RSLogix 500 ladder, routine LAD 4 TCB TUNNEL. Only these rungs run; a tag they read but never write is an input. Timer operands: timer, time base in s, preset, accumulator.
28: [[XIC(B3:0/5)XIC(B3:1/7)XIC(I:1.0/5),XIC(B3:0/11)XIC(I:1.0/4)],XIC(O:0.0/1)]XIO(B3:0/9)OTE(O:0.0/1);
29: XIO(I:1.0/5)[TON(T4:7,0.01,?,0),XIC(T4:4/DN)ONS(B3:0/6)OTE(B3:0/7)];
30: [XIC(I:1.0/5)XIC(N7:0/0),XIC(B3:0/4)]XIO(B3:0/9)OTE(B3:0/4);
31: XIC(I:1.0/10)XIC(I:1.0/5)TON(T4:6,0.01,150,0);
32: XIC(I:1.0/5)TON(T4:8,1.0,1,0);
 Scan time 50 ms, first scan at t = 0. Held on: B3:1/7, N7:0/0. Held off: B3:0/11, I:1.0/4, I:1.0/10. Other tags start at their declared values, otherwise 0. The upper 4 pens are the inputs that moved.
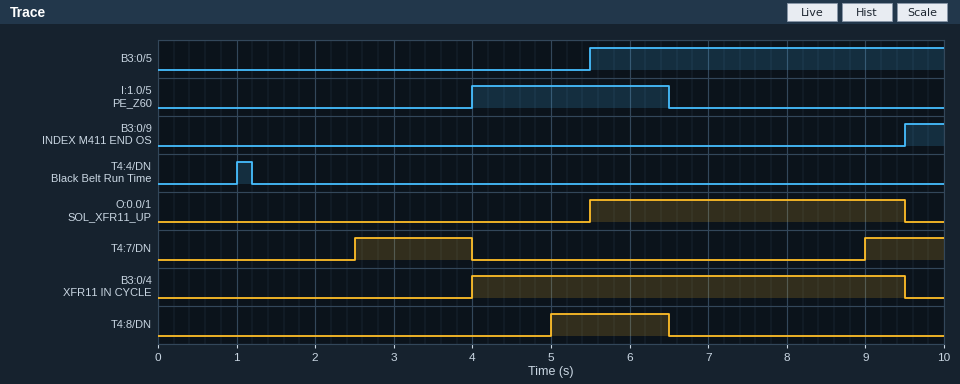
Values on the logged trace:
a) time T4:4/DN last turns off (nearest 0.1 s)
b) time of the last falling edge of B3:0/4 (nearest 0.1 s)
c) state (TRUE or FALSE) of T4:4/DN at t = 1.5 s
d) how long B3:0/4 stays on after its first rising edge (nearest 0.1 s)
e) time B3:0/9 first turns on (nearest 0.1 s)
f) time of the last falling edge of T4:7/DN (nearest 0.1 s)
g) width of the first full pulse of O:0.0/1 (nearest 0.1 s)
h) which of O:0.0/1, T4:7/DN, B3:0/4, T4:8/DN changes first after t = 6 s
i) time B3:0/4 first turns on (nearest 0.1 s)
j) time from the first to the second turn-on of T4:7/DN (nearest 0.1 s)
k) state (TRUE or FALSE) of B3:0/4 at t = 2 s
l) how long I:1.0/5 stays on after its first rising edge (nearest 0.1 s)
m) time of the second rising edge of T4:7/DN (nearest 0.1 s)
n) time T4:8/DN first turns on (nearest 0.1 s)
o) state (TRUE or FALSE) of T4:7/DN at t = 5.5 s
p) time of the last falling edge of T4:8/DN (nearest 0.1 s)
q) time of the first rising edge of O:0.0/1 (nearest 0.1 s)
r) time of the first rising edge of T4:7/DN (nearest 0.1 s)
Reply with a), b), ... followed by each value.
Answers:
a) 1.2 s
b) 9.5 s
c) FALSE
d) 5.5 s
e) 9.5 s
f) 4.0 s
g) 4.0 s
h) T4:8/DN
i) 4.0 s
j) 6.5 s
k) FALSE
l) 2.5 s
m) 9.0 s
n) 5.0 s
o) FALSE
p) 6.5 s
q) 5.5 s
r) 2.5 s
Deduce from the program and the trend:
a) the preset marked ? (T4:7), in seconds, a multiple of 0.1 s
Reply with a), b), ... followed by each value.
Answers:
a) 2.5 s
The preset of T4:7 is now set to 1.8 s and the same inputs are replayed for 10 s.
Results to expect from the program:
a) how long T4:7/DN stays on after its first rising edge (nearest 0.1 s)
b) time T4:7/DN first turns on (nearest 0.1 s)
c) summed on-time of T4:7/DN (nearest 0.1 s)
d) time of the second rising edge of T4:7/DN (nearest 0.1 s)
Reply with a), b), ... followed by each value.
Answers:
a) 2.2 s
b) 1.8 s
c) 3.9 s
d) 8.3 s
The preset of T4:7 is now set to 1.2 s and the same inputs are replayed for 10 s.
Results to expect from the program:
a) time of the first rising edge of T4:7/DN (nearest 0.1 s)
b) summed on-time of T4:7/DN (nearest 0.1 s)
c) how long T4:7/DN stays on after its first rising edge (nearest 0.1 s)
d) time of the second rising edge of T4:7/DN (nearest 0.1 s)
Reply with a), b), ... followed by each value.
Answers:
a) 1.2 s
b) 5.1 s
c) 2.8 s
d) 7.7 s
